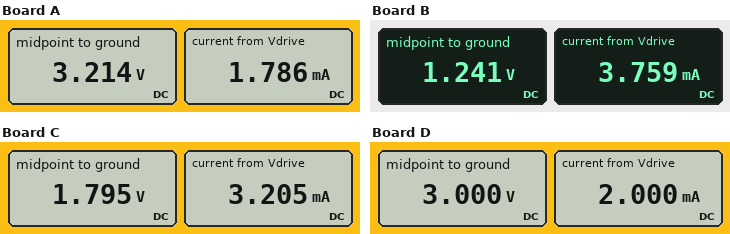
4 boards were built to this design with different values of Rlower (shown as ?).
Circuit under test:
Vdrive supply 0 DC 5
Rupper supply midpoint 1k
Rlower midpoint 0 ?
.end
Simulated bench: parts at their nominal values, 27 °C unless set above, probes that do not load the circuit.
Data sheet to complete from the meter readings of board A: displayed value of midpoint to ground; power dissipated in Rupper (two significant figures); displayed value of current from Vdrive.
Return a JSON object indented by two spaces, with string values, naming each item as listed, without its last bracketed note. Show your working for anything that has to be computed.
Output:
{
  "displayed value of midpoint to ground": "3.214 V",
  "power dissipated in Rupper": "(5 V - 3.214 V)^2 / 1 kΩ = 3.2 mW",
  "displayed value of current from Vdrive": "1.786 mA"
}
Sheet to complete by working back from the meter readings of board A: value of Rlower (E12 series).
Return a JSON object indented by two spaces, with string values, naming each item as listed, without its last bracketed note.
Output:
{
  "value of Rlower": "1.8 kΩ"
}
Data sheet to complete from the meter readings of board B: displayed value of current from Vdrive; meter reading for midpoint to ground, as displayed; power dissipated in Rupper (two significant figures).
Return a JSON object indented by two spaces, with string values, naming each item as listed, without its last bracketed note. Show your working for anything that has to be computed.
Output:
{
  "displayed value of current from Vdrive": "3.759 mA",
  "meter reading for midpoint to ground, as displayed": "1.241 V",
  "power dissipated in Rupper": "(5 V - 1.241 V)^2 / 1 kΩ = 14 mW"
}
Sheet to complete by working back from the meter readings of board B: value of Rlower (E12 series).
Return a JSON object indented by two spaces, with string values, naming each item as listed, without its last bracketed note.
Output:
{
  "value of Rlower": "330 Ω"
}
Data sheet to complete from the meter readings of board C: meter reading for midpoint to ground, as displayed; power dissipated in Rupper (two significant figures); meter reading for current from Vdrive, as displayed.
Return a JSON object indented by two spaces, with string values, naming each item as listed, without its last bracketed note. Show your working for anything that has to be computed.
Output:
{
  "meter reading for midpoint to ground, as displayed": "1.795 V",
  "power dissipated in Rupper": "(5 V - 1.795 V)^2 / 1 kΩ = 10 mW",
  "meter reading for current from Vdrive, as displayed": "3.205 mA"
}
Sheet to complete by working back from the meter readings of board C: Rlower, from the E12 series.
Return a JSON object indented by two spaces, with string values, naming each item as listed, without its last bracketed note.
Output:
{
  "Rlower, from the E12 series": "560 Ω"
}
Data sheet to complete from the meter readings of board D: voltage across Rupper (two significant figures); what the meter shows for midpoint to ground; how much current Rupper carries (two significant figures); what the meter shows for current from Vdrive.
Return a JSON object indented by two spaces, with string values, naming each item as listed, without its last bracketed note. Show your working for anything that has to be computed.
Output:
{
  "voltage across Rupper": "5 V - 3 V = 2.0 V",
  "what the meter shows for midpoint to ground": "3.000 V",
  "how much current Rupper carries": "(5 V - 3 V) / 1 kΩ = 2.0 mA",
  "what the meter shows for current from Vdrive": "2.000 mA"
}
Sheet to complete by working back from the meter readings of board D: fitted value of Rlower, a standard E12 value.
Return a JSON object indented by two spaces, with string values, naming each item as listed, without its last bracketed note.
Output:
{
  "fitted value of Rlower, a standard E12 value": "1.5 kΩ"
}
